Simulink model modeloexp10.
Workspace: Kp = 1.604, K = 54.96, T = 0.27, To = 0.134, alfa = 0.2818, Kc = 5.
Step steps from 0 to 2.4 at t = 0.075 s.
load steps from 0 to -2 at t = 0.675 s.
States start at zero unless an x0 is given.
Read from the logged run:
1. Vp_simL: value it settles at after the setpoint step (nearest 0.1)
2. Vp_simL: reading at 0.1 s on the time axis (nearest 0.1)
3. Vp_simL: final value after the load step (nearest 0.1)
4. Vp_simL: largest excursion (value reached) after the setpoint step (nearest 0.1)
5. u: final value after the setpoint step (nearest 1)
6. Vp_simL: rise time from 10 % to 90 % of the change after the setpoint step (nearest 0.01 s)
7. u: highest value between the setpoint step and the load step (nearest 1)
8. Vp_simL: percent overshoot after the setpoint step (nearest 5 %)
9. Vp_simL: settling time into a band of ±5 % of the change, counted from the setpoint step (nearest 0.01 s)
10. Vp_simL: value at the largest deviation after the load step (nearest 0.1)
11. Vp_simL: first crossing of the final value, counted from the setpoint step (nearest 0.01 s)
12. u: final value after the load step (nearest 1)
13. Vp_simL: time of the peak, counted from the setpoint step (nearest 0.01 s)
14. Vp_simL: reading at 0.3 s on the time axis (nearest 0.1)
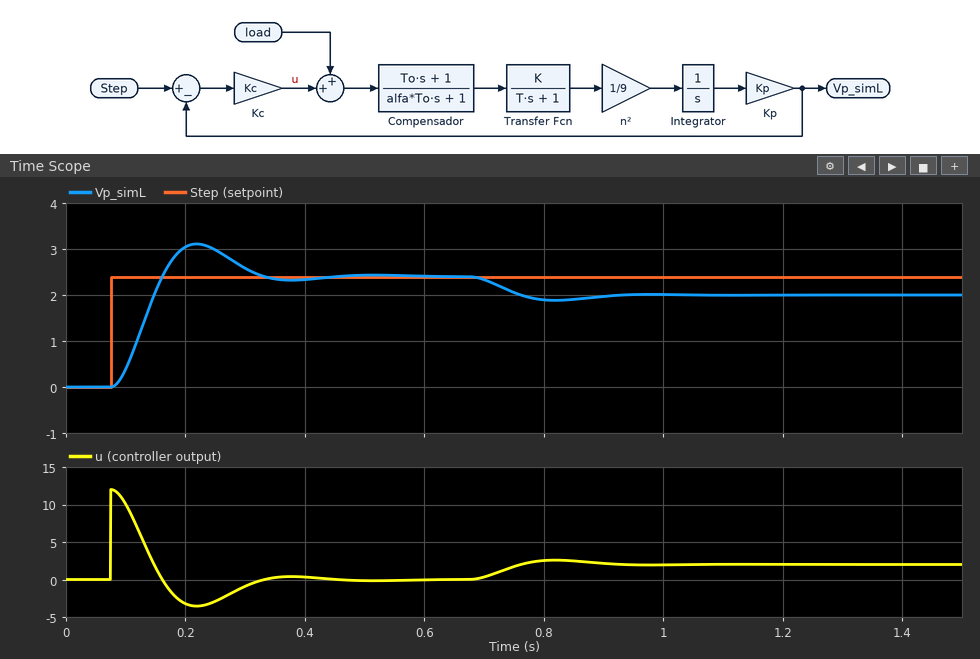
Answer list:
2.4
0.4
2.0
3.1
0
0.06 s
12
30 %
0.23 s
1.9
0.09 s
2
0.14 s
2.6
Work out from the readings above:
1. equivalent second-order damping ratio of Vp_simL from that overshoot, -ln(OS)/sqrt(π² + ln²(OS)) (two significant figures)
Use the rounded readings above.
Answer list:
0.36
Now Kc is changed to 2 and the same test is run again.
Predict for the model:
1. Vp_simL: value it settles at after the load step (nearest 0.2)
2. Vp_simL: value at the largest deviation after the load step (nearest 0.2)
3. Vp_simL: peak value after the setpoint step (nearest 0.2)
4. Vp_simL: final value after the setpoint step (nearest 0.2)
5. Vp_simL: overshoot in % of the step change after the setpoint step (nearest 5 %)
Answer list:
1.4
1.2
2.8
2.4
20 %
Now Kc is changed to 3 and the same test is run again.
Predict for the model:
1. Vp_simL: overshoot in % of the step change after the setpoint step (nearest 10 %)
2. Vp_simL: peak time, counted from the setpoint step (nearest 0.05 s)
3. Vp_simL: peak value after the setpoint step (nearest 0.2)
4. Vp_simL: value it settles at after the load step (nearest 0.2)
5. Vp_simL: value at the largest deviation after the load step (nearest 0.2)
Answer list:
20 %
0.20 s
3.0
1.8
1.6
